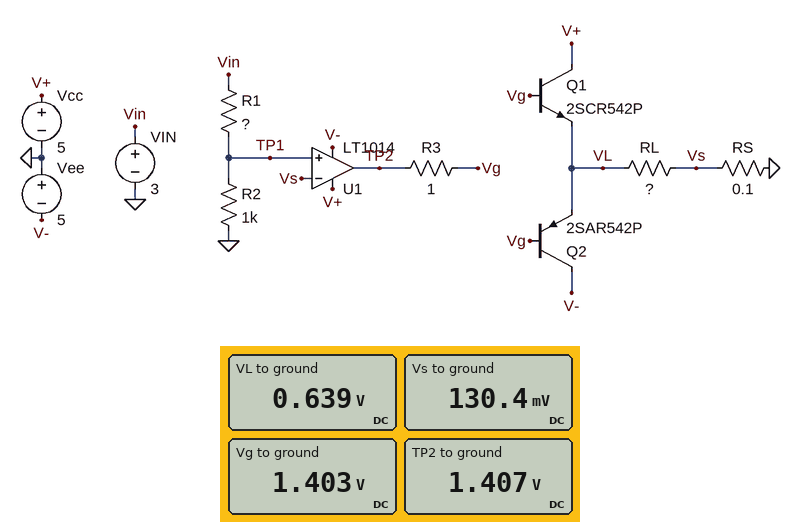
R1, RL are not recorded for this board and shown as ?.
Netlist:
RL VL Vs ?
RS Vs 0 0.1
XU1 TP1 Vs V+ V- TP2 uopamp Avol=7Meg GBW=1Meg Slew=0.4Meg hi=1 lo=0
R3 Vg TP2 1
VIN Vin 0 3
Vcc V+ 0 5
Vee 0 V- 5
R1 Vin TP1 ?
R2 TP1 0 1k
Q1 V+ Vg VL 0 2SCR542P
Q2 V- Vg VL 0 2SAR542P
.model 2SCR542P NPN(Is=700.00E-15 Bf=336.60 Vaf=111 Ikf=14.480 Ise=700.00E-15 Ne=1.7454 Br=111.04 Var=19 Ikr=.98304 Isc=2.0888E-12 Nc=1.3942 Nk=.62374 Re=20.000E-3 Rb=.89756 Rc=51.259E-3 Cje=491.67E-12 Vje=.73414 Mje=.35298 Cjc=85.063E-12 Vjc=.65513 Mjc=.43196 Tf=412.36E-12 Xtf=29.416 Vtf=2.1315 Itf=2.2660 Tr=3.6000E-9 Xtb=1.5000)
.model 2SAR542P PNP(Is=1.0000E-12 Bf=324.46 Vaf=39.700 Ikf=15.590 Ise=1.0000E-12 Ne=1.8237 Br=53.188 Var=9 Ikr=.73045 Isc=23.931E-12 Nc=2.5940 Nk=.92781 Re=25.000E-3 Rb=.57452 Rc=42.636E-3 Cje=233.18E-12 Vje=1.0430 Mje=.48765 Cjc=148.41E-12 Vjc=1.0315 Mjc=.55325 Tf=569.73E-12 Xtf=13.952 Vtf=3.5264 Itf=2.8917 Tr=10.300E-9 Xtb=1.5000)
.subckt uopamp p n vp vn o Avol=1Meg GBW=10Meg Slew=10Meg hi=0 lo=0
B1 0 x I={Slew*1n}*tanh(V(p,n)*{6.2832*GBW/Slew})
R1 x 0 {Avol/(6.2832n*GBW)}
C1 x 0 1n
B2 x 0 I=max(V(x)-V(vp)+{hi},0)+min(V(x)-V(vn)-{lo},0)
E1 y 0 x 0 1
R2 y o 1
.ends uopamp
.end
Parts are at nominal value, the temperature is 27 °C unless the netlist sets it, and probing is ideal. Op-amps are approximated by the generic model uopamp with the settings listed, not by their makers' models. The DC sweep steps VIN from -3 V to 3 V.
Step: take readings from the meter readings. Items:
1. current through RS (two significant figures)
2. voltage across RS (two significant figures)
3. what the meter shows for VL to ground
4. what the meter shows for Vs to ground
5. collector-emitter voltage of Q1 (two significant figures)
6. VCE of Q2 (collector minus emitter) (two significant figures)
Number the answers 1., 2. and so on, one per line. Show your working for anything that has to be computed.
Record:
1. (130.4 mV) / 100 mΩ = 1.3 A
2. 130.4 mV = 130 mV
3. 0.639 V
4. 130.4 mV
5. 5 V - 639 mV = 4.4 V
6. -5 V - 639 mV = -5.6 V
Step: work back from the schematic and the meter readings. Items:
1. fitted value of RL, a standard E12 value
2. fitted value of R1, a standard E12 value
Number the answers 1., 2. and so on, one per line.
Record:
1. 0.39 Ω
2. 22 kΩ
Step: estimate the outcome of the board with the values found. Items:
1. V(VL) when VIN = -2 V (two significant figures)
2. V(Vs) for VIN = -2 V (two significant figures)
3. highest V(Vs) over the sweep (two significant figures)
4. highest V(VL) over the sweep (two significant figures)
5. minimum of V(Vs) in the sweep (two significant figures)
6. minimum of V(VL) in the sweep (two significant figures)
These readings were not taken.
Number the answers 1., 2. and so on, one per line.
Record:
1. -430 mV
2. -87 mV
3. 130 mV
4. 640 mV
5. -130 mV
6. -640 mV
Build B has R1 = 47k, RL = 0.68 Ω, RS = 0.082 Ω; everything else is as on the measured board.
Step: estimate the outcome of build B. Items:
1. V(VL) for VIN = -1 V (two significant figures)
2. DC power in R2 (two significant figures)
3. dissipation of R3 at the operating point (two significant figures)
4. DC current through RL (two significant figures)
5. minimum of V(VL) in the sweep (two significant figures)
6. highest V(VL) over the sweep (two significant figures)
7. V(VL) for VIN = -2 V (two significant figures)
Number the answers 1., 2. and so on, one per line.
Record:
1. -190 mV
2. 3.9 µW
3. 5.9 µW
4. 760 mA
5. -580 mV
6. 580 mV
7. -390 mV
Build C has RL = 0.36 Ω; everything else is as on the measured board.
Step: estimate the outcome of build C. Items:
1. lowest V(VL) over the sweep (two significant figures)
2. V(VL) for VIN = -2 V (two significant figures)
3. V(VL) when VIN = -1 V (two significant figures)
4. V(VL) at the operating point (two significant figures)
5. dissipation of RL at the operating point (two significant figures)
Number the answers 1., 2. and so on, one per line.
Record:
1. -600 mV
2. -400 mV
3. -200 mV
4. 600 mV
5. 610 mW
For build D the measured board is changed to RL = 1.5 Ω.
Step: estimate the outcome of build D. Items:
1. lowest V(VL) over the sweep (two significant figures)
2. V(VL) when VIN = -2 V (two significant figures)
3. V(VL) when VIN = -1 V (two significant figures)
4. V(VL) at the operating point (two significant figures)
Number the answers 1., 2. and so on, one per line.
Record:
1. -2.1 V
2. -1.4 V
3. -700 mV
4. 2.1 V
